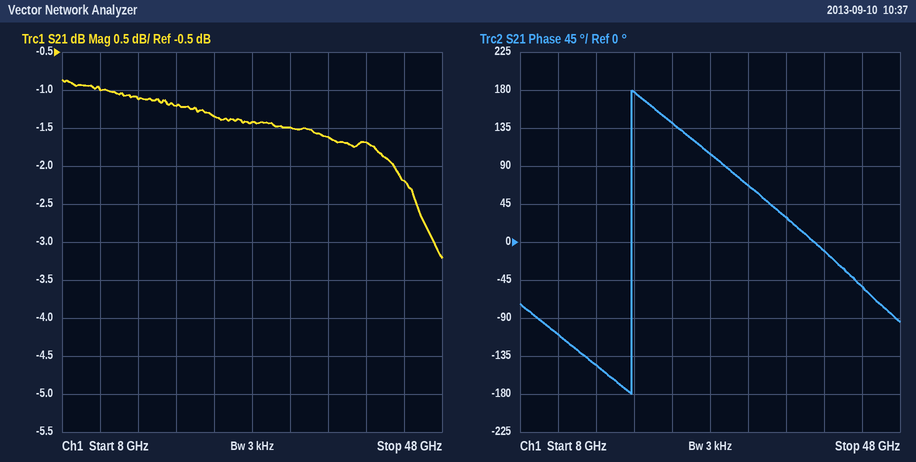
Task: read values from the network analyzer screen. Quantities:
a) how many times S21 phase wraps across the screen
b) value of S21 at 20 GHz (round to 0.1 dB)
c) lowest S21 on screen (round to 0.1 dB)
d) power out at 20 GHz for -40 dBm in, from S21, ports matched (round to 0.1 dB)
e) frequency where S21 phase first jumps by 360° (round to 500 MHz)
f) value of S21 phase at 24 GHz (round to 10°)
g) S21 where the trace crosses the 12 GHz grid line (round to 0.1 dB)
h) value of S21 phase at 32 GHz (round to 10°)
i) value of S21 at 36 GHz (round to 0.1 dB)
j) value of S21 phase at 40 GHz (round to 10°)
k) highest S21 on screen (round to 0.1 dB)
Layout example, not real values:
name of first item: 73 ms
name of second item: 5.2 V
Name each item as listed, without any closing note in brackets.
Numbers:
how many times S21 phase wraps across the screen: 1
value of S21 at 20 GHz: -1.2 dB
lowest S21 on screen: -3.2 dB
power out at 20 GHz for -40 dBm in, from S21, ports matched: -41.2 dBm
frequency where S21 phase first jumps by 360°: 19.5 GHz
value of S21 phase at 24 GHz: 140°
S21 where the trace crosses the 12 GHz grid line: -1.0 dB
value of S21 phase at 32 GHz: 70°
value of S21 at 36 GHz: -1.6 dB
value of S21 phase at 40 GHz: -10°
highest S21 on screen: -0.9 dB
